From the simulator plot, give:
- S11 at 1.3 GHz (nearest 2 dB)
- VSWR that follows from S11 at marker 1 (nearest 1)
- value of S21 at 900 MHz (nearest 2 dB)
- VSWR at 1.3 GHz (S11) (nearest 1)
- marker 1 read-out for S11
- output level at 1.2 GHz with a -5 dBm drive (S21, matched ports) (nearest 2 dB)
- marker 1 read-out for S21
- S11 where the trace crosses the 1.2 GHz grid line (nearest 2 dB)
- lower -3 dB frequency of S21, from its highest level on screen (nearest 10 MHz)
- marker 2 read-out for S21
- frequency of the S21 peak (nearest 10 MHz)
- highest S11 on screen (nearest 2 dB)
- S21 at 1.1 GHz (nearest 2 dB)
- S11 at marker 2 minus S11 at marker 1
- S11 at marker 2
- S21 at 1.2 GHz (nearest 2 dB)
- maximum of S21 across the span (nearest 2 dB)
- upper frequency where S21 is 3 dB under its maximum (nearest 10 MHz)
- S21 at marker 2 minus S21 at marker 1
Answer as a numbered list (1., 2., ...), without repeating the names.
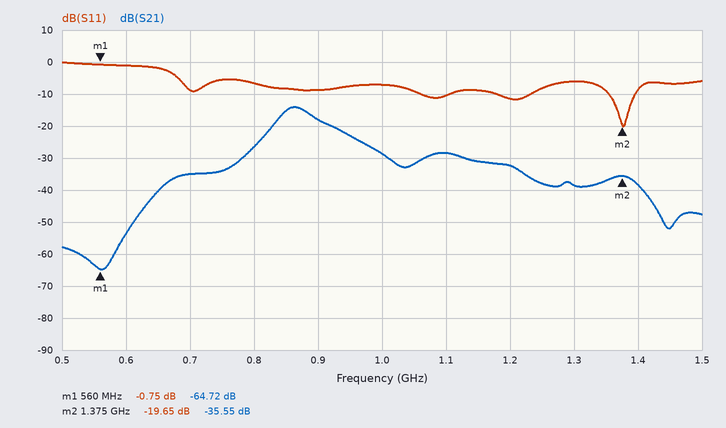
1. -6 dB
2. 23
3. -18 dB
4. 3
5. -0.75 dB
6. -38 dBm
7. -64.72 dB
8. -12 dB
9. 840 MHz
10. -35.55 dB
11. 860 MHz
12. 0 dB
13. -28 dB
14. -18.90 dB
15. -19.65 dB
16. -32 dB
17. -14 dB
18. 890 MHz
19. 29.17 dB
